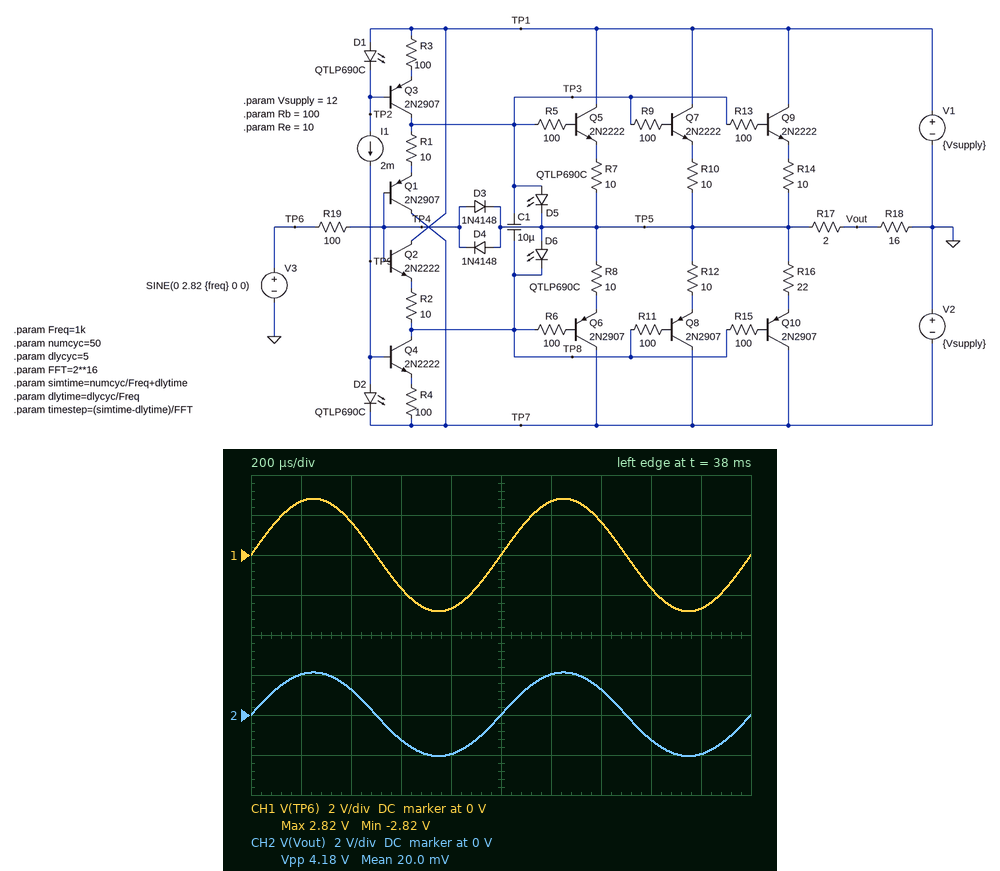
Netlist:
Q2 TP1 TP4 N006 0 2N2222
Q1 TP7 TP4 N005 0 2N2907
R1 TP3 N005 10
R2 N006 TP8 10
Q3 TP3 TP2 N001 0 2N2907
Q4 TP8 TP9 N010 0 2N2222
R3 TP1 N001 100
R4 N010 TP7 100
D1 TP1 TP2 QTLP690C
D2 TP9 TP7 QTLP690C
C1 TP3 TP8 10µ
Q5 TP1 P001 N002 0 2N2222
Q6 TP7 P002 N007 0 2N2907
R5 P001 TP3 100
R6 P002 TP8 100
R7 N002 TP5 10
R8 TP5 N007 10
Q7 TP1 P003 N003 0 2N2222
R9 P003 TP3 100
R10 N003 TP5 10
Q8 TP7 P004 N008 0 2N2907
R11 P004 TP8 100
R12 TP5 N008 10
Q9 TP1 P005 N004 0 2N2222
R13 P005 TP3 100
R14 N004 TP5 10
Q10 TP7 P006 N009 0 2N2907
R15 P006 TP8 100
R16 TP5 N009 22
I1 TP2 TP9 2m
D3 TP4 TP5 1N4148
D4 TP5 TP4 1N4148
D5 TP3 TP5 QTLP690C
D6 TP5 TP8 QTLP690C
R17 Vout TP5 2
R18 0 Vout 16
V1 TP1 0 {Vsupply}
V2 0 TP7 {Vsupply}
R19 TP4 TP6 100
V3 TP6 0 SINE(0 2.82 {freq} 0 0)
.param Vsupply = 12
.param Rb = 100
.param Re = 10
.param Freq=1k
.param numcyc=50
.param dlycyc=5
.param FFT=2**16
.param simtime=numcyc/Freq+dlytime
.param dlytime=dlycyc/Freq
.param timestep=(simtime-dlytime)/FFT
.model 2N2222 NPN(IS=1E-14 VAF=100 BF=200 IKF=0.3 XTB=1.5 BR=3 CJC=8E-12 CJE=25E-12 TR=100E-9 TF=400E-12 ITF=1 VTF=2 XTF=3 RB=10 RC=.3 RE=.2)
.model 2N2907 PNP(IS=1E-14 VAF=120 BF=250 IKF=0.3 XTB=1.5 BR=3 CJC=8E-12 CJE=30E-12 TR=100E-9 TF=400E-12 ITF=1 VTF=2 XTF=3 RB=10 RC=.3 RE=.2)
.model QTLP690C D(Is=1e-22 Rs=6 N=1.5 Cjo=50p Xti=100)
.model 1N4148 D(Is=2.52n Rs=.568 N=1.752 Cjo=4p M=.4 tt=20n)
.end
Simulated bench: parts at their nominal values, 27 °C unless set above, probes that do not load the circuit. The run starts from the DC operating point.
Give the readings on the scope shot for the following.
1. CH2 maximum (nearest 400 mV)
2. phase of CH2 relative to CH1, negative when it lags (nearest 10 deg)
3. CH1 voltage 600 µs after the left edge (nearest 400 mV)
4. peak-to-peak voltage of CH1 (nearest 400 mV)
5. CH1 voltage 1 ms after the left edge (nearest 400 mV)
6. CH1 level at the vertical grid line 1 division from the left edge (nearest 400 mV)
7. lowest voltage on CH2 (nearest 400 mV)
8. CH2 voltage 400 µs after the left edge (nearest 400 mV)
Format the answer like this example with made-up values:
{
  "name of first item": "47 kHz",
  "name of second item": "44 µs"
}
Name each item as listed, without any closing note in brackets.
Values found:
{
  "CH2 maximum": "2.0 V",
  "phase of CH2 relative to CH1, negative when it lags": "0 deg",
  "CH1 voltage 600 µs after the left edge": "-1.6 V",
  "peak-to-peak voltage of CH1": "5.6 V",
  "CH1 voltage 1 ms after the left edge": "0 V",
  "CH1 level at the vertical grid line 1 division from the left edge": "2.8 V",
  "lowest voltage on CH2": "-2.0 V",
  "CH2 voltage 400 µs after the left edge": "1.2 V"
}
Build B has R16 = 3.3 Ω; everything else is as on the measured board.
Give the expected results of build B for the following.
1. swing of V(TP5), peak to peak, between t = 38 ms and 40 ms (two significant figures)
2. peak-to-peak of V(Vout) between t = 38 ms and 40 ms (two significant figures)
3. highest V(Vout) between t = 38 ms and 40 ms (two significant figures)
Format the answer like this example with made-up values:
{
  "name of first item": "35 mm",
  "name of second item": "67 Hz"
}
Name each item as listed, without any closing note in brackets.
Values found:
{
  "swing of V(TP5), peak to peak, between t = 38 ms and 40 ms": "4.9 V",
  "peak-to-peak of V(Vout) between t = 38 ms and 40 ms": "4.4 V",
  "highest V(Vout) between t = 38 ms and 40 ms": "2.1 V"
}
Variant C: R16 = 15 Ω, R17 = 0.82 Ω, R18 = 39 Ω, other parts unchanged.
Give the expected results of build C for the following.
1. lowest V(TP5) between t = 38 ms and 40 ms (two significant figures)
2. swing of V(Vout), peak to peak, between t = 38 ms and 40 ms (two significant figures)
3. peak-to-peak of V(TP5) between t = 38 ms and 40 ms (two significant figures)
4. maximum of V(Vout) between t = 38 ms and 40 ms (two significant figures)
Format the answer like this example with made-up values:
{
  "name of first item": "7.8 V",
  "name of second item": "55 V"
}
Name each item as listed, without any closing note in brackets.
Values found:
{
  "lowest V(TP5) between t = 38 ms and 40 ms": "-2.6 V",
  "swing of V(Vout), peak to peak, between t = 38 ms and 40 ms": "5.2 V",
  "peak-to-peak of V(TP5) between t = 38 ms and 40 ms": "5.3 V",
  "maximum of V(Vout) between t = 38 ms and 40 ms": "2.6 V"
}
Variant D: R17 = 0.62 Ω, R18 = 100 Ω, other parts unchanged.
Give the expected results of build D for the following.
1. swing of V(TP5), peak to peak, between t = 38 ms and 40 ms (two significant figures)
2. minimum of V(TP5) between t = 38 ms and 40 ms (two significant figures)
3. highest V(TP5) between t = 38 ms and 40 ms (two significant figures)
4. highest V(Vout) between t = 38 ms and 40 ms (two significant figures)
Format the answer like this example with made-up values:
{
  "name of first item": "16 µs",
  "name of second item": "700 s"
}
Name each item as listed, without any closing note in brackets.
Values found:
{
  "swing of V(TP5), peak to peak, between t = 38 ms and 40 ms": "5.5 V",
  "minimum of V(TP5) between t = 38 ms and 40 ms": "-2.7 V",
  "highest V(TP5) between t = 38 ms and 40 ms": "2.8 V",
  "highest V(Vout) between t = 38 ms and 40 ms": "2.7 V"
}
